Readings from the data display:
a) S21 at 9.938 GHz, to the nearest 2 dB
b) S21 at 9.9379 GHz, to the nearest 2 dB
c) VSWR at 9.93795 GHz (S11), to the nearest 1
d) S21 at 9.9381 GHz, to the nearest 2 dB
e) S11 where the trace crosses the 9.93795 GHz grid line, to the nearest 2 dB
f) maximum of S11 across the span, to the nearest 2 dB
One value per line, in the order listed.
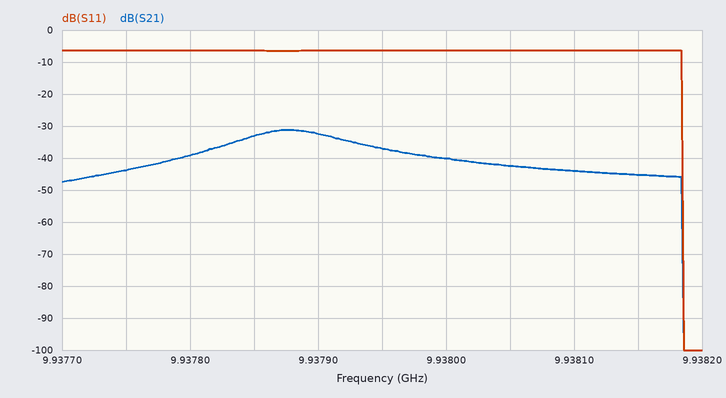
-40 dB
-32 dB
3
-44 dB
-6 dB
-6 dB
